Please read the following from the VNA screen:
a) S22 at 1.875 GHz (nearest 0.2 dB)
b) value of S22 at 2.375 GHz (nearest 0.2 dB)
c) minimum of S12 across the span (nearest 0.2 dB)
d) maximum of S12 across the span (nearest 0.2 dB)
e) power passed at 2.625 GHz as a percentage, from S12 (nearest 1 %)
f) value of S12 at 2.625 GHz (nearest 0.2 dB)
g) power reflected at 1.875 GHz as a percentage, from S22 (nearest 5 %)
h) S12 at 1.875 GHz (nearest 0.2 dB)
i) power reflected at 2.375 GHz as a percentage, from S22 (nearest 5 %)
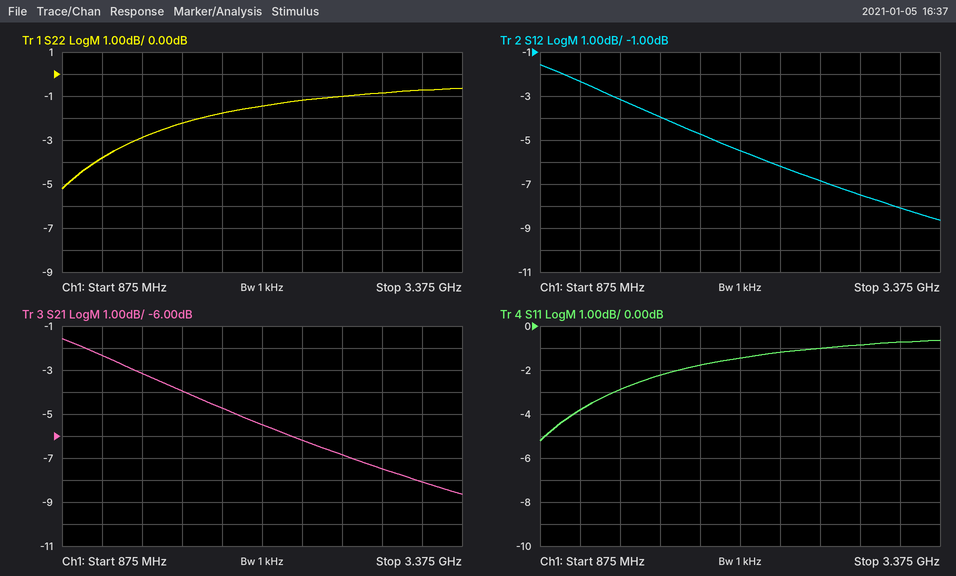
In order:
-1.8 dB
-1.2 dB
-8.6 dB
-1.6 dB
21 %
-6.8 dB
65 %
-4.8 dB
75 %
